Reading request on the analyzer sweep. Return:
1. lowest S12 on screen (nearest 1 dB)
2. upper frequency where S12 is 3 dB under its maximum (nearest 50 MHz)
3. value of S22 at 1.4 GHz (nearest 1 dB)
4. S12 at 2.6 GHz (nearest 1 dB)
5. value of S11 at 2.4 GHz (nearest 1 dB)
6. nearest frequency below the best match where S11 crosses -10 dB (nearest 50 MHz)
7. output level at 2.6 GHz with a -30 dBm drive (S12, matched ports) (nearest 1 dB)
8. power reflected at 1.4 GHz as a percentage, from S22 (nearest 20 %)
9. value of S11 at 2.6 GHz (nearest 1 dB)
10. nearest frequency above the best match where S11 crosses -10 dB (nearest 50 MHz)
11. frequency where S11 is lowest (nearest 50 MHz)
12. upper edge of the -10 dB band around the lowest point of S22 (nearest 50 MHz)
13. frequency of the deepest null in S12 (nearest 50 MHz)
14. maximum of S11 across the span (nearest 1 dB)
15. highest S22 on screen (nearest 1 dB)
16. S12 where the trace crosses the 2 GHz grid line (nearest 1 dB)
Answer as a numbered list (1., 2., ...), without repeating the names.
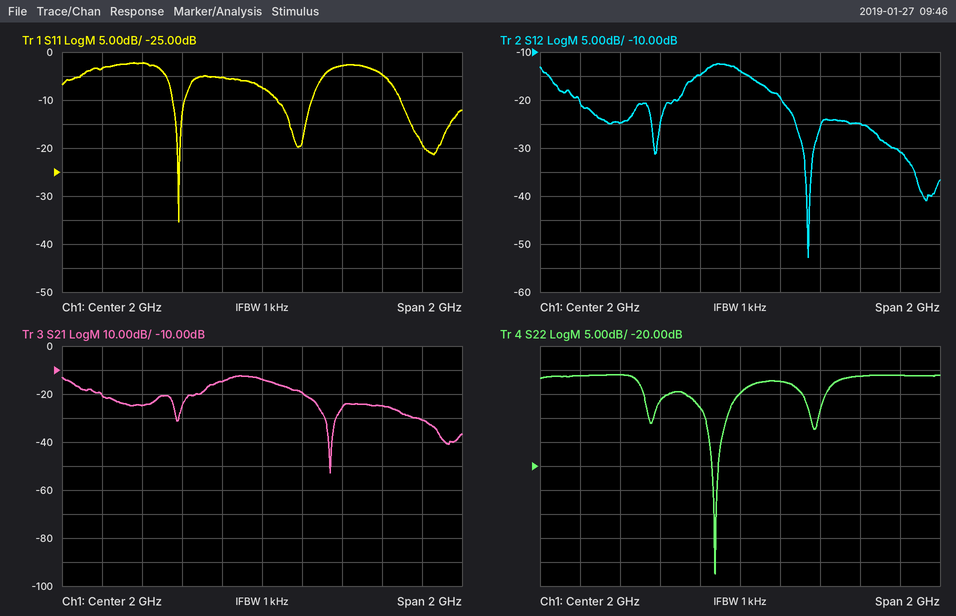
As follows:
1. -53 dB
2. 2.05 GHz
3. -1 dB
4. -25 dB
5. -3 dB
6. 1.55 GHz
7. -55 dBm
8. 80 %
9. -5 dB
10. 1.60 GHz
11. 1.60 GHz
12. 1.95 GHz
13. 2.35 GHz
14. -2 dB
15. -1 dB
16. -14 dB
